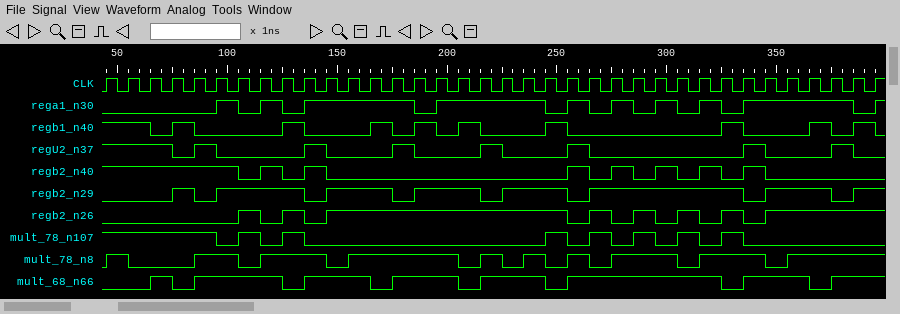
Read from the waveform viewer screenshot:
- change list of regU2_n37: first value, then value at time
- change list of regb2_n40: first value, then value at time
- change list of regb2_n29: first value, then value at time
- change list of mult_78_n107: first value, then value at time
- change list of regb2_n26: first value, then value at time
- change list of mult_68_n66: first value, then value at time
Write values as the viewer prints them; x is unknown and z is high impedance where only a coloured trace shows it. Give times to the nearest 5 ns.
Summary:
1, 0 at 75 ns, 1 at 85 ns, 0 at 95 ns, 1 at 135 ns, 0 at 145 ns, 1 at 175 ns, 0 at 185 ns, 1 at 215 ns, 0 at 225 ns, 1 at 255 ns, 0 at 265 ns, 1 at 335 ns, 0 at 345 ns, 1 at 375 ns, 0 at 385 ns
1, 0 at 105 ns, 1 at 115 ns, 0 at 125 ns, 1 at 135 ns, 0 at 145 ns, 1 at 255 ns, 0 at 265 ns, 1 at 275 ns, 0 at 285 ns, 1 at 295 ns, 0 at 305 ns, 1 at 315 ns, 0 at 325 ns, 1 at 335 ns, 0 at 345 ns
0, 1 at 75 ns, 0 at 85 ns, 1 at 95 ns, 0 at 135 ns, 1 at 145 ns, 0 at 175 ns, 1 at 185 ns, 0 at 215 ns, 1 at 225 ns, 0 at 255 ns, 1 at 265 ns, 0 at 335 ns, 1 at 345 ns, 0 at 375 ns, 1 at 385 ns
1, 0 at 95 ns, 1 at 105 ns, 0 at 115 ns, 1 at 125 ns, 0 at 135 ns, 1 at 245 ns, 0 at 255 ns, 1 at 265 ns, 0 at 275 ns, 1 at 285 ns, 0 at 295 ns, 1 at 305 ns, 0 at 315 ns, 1 at 325 ns, 0 at 335 ns
0, 1 at 105 ns, 0 at 115 ns, 1 at 125 ns, 0 at 135 ns, 1 at 145 ns, 0 at 255 ns, 1 at 265 ns, 0 at 275 ns, 1 at 285 ns, 0 at 295 ns, 1 at 305 ns, 0 at 315 ns, 1 at 325 ns, 0 at 335 ns, 1 at 345 ns
0, 1 at 65 ns, 0 at 75 ns, 1 at 85 ns, 0 at 125 ns, 1 at 135 ns, 0 at 165 ns, 1 at 175 ns, 0 at 205 ns, 1 at 215 ns, 0 at 245 ns, 1 at 255 ns, 0 at 325 ns, 1 at 335 ns, 0 at 365 ns, 1 at 375 ns
